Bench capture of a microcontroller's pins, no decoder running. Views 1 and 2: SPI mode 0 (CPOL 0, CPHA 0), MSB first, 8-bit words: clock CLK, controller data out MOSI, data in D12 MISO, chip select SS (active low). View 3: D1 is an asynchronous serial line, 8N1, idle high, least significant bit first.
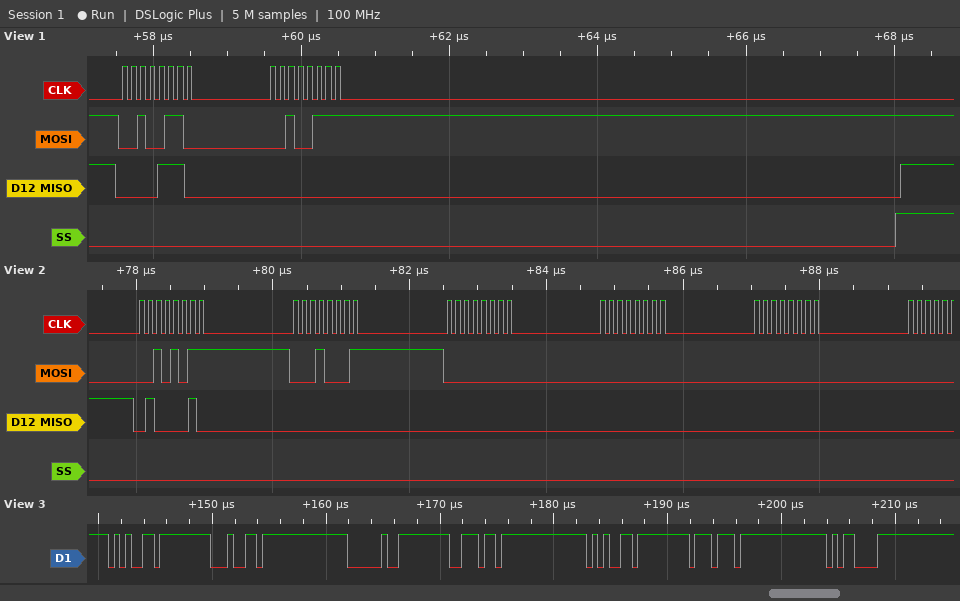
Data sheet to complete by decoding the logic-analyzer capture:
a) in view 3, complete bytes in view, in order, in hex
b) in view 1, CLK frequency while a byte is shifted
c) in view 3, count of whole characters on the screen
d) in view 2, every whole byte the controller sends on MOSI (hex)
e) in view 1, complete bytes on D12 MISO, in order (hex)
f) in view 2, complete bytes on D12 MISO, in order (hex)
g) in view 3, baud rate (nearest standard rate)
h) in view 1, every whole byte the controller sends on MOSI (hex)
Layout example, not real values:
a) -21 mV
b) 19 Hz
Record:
a) 65 64 20 6E 65 77 0D
b) 8 MHz
c) 7
d) 2B 11 00 00 00
e) 0E 00
f) 42 00 00 00 00
g) 2000000 baud
h) 26 27
